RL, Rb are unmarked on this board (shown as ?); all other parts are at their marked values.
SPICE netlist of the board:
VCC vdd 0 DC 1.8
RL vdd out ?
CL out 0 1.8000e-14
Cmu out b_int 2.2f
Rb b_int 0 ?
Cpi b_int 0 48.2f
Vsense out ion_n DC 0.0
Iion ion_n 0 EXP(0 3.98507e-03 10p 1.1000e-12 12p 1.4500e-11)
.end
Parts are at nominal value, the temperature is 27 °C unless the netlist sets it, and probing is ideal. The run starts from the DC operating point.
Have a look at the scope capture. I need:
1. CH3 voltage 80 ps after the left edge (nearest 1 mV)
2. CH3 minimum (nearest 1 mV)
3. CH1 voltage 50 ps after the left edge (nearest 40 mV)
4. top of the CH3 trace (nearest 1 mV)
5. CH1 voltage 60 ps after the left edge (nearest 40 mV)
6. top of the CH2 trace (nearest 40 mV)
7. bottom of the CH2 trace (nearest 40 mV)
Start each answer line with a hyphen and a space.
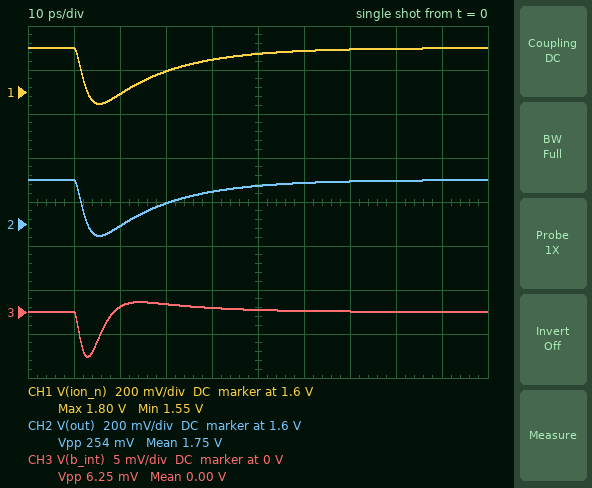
- 0 V
- -5 mV
- 1.76 V
- 1 mV
- 1.80 V
- 1.80 V
- 1.56 V
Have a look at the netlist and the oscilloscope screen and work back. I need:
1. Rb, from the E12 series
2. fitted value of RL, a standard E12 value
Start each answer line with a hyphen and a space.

- 47 Ω
- 82 Ω
